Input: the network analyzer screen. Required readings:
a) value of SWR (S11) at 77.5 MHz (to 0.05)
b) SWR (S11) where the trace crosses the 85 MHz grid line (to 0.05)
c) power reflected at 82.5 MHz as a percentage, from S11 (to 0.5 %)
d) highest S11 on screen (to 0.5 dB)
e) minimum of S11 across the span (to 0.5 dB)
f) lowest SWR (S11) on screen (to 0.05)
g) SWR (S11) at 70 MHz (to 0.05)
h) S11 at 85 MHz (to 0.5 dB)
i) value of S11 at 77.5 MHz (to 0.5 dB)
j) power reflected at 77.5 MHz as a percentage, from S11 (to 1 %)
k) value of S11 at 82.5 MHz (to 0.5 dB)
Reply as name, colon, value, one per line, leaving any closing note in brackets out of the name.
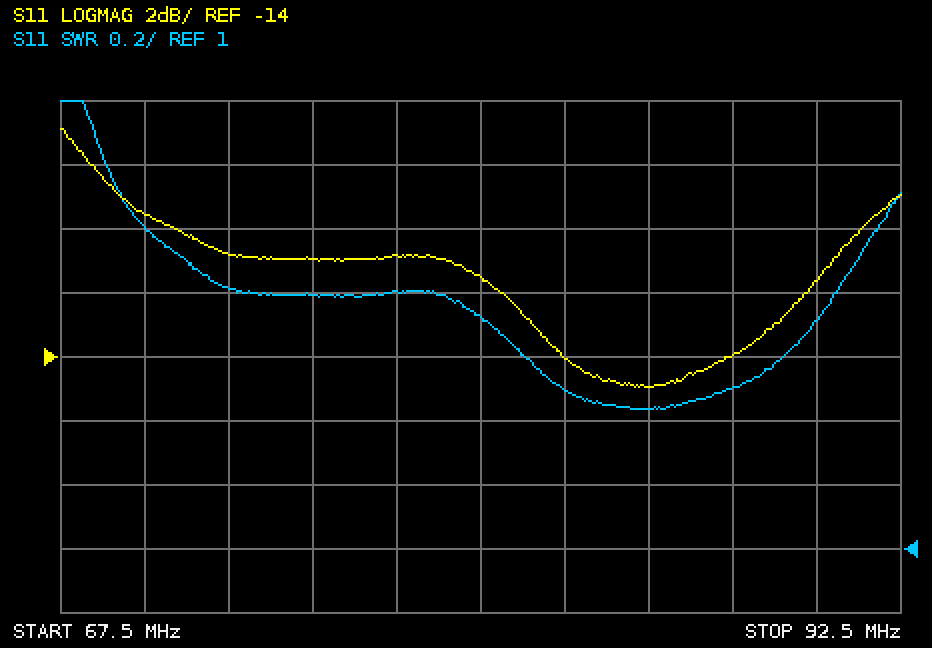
value of SWR (S11) at 77.5 MHz: 1.80
SWR (S11) where the trace crosses the 85 MHz grid line: 1.45
power reflected at 82.5 MHz as a percentage, from S11: 4.0 %
highest S11 on screen: -7.0 dB
minimum of S11 across the span: -15.0 dB
lowest SWR (S11) on screen: 1.45
SWR (S11) at 70 MHz: 2.00
S11 at 85 MHz: -15.0 dB
value of S11 at 77.5 MHz: -11.0 dB
power reflected at 77.5 MHz as a percentage, from S11: 8 %
value of S11 at 82.5 MHz: -14.0 dB
